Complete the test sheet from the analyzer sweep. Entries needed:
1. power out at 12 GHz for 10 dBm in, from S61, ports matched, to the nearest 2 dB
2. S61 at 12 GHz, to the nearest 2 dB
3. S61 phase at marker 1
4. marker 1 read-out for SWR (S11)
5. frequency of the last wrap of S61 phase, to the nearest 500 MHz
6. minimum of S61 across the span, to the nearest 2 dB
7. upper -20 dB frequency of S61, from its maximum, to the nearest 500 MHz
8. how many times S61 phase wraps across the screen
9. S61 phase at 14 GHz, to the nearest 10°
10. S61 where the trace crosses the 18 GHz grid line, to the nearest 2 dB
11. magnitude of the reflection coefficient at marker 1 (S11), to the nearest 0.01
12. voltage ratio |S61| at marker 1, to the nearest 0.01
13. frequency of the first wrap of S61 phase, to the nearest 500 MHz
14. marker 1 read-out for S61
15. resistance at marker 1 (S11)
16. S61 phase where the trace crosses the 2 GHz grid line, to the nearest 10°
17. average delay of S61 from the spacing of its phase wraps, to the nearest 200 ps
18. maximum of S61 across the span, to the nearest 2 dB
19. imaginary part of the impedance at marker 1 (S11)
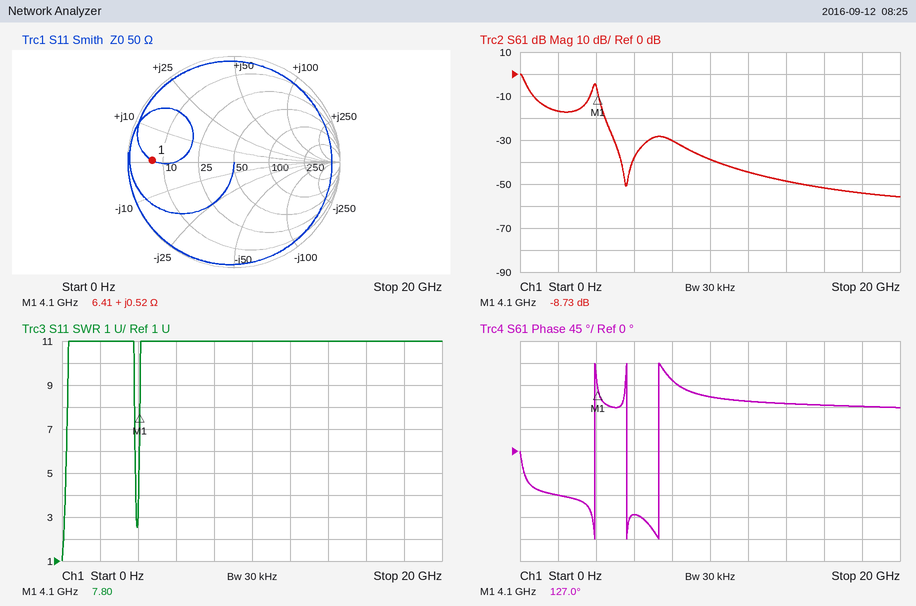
-34 dBm
-44 dB
127.0°
7.80
7.5 GHz
-56 dB
4.5 GHz
3
100°
-54 dB
0.77
0.37
4.0 GHz
-8.73 dB
6.41 Ω
-90°
600 ps
0 dB
+0.52 Ω
